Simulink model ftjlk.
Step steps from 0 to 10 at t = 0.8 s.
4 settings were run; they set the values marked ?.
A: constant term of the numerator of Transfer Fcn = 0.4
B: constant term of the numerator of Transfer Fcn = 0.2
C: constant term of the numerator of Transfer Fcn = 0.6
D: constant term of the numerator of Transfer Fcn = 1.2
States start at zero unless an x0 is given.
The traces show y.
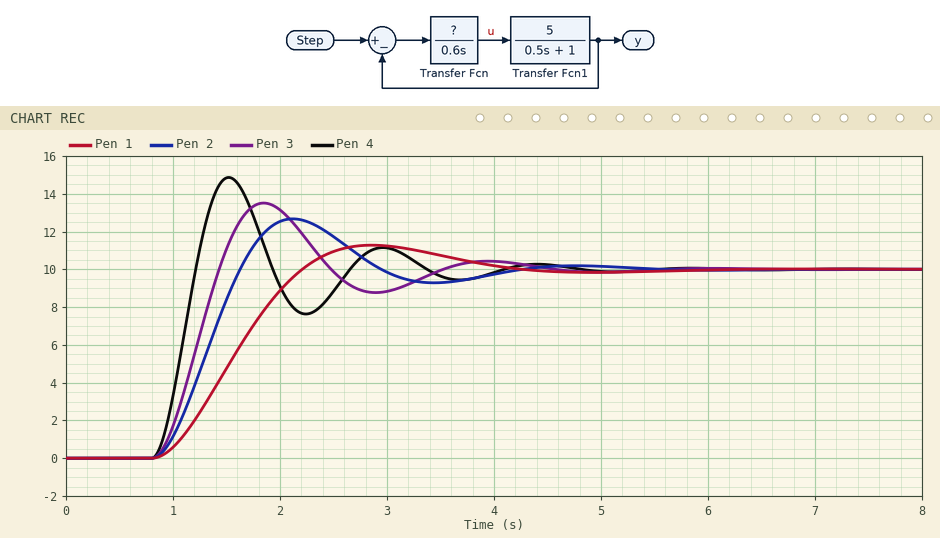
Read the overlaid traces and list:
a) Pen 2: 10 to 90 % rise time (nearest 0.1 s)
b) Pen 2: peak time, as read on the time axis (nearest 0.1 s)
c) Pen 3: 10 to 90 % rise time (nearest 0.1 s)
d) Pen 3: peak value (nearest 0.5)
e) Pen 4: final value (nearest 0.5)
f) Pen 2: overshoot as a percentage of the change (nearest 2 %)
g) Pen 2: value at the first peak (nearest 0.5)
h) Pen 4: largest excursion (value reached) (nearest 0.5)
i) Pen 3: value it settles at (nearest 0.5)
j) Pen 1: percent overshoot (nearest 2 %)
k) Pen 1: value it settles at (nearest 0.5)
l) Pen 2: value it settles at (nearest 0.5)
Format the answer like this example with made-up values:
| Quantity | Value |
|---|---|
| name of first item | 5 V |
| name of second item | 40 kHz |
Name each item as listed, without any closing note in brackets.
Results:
| Quantity | Value |
|---|---|
| Pen 2: 10 to 90 % rise time | 0.6 s |
| Pen 2: peak time, as read on the time axis | 2.1 s |
| Pen 3: 10 to 90 % rise time | 0.4 s |
| Pen 3: peak value | 13.5 |
| Pen 4: final value | 10.0 |
| Pen 2: overshoot as a percentage of the change | 26 % |
| Pen 2: value at the first peak | 12.5 |
| Pen 4: largest excursion (value reached) | 15.0 |
| Pen 3: value it settles at | 10.0 |
| Pen 1: percent overshoot | 12 % |
| Pen 1: value it settles at | 10.0 |
| Pen 2: value it settles at | 10.0 |
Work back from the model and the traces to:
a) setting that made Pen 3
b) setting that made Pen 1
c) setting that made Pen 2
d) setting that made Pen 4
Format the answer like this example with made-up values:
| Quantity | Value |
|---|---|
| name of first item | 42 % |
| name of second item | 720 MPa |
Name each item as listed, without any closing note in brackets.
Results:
| Quantity | Value |
|---|---|
| setting that made Pen 3 | C |
| setting that made Pen 1 | B |
| setting that made Pen 2 | A |
| setting that made Pen 4 | D |
